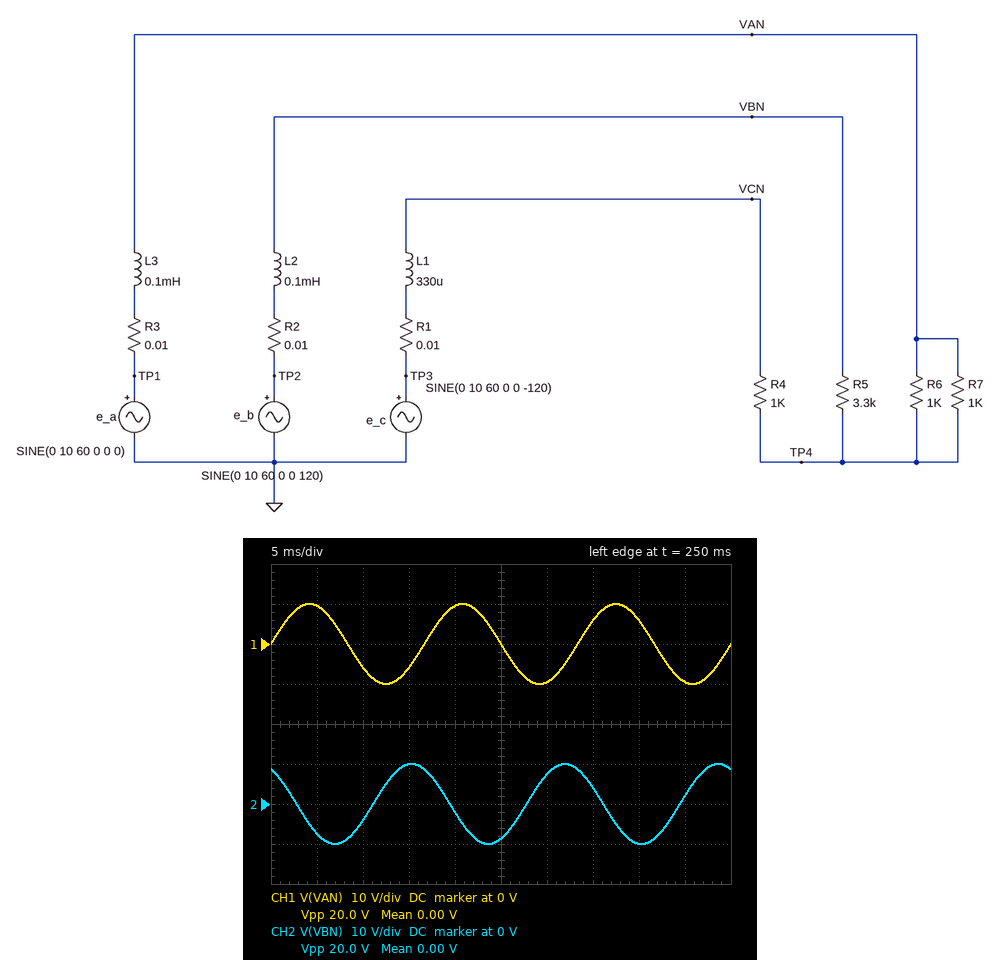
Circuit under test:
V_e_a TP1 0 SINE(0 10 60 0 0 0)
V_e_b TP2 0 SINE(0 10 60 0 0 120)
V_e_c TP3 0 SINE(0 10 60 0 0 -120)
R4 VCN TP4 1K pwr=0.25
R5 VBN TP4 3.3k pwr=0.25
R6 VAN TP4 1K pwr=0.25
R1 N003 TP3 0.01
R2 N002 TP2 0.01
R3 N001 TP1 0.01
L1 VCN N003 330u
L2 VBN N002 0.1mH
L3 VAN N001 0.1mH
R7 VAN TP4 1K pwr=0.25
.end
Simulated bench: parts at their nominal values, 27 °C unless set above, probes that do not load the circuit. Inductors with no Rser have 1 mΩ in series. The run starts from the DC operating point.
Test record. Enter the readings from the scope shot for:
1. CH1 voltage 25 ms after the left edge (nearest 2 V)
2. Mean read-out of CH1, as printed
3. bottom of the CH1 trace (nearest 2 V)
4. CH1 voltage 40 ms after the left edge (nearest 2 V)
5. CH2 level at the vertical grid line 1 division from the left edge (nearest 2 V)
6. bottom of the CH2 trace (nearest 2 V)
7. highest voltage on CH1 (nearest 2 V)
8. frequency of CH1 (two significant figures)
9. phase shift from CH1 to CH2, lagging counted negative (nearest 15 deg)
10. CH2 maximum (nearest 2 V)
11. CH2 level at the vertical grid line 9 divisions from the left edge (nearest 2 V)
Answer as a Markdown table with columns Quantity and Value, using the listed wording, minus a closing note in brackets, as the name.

| Quantity | Value |
|---|---|
| CH1 voltage 25 ms after the left edge | 0 V |
| Mean read-out of CH1, as printed | 0.00 V |
| bottom of the CH1 trace | -10 V |
| CH1 voltage 40 ms after the left edge | 6 V |
| CH2 level at the vertical grid line 1 division from the left edge | -8 V |
| bottom of the CH2 trace | -10 V |
| highest voltage on CH1 | 10 V |
| frequency of CH1 | 60 Hz |
| phase shift from CH1 to CH2, lagging counted negative | 120 deg |
| CH2 maximum | 10 V |
| CH2 level at the vertical grid line 9 divisions from the left edge | 2 V |
